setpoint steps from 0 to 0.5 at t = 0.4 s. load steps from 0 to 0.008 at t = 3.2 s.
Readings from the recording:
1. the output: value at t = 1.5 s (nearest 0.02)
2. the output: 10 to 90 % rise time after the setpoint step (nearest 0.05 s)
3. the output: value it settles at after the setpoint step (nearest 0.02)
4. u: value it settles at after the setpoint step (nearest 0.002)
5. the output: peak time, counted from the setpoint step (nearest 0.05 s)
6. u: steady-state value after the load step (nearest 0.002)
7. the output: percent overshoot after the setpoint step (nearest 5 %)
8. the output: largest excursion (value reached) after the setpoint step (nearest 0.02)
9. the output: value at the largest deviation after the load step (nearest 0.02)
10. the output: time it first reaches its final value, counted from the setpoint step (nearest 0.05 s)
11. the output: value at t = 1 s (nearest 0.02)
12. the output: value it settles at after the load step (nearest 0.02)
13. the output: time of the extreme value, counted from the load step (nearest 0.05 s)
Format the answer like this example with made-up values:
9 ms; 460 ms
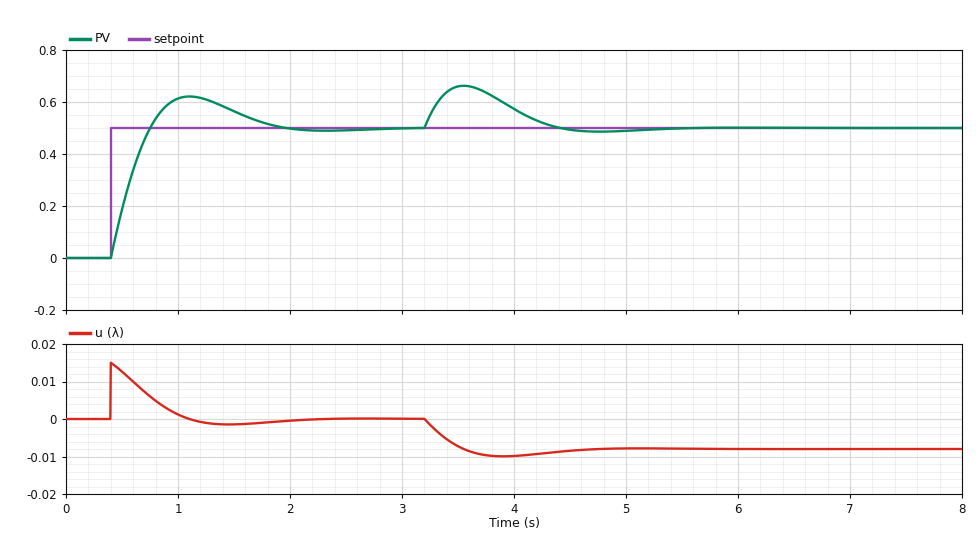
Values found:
0.56; 0.25 s; 0.50; 0.000; 0.70 s; -0.008; 25 %; 0.62; 0.66; 0.35 s; 0.62; 0.50; 0.35 s
